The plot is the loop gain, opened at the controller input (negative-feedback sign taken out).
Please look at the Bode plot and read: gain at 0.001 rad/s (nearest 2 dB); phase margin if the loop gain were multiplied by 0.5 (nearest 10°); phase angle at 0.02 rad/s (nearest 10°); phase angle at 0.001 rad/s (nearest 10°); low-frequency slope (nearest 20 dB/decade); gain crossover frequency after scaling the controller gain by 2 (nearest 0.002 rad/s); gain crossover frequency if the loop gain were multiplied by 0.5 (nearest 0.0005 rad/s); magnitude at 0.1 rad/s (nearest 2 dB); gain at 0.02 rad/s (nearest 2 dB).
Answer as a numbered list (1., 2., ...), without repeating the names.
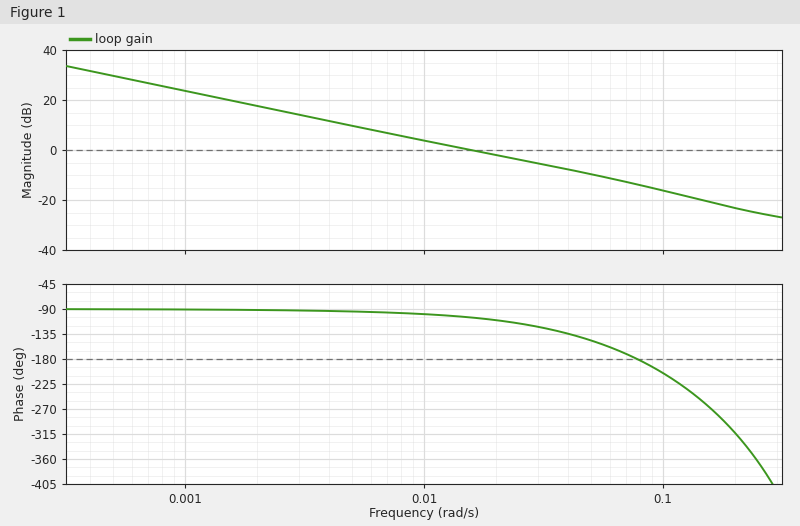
1. 24 dB
2. 80°
3. -110°
4. -90°
5. -20 dB/decade
6. 0.032 rad/s
7. 0.0075 rad/s
8. -16 dB
9. -2 dB
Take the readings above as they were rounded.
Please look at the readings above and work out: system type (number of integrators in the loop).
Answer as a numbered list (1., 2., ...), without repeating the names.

1. 1
